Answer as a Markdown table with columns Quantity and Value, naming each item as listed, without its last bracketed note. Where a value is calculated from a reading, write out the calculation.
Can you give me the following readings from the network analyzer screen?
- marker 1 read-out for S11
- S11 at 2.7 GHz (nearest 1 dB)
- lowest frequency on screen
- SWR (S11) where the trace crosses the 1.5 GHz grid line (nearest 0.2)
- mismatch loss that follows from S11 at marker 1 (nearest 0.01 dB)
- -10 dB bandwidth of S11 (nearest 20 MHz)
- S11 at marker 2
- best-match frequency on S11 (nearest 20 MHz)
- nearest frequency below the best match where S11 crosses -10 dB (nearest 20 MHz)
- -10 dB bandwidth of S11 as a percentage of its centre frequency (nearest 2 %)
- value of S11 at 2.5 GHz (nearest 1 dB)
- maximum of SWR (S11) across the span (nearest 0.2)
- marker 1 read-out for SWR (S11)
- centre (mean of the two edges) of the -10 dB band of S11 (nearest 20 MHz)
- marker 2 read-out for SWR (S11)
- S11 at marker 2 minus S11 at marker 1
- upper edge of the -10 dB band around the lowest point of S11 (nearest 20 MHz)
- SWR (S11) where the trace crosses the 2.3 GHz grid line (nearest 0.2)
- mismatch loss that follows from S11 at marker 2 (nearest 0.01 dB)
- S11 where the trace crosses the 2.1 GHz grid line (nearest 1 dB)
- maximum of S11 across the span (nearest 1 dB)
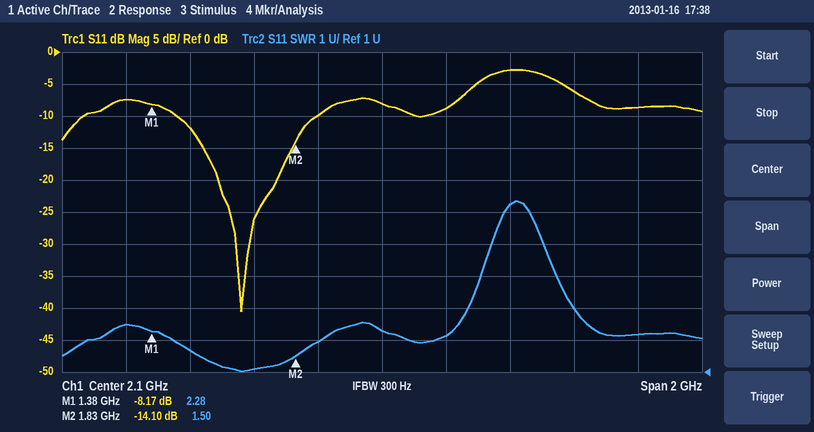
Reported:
| Quantity | Value |
|---|---|
| marker 1 read-out for S11 | -8.17 dB |
| S11 at 2.7 GHz | -6 dB |
| lowest frequency on screen | 1.1 GHz |
| SWR (S11) where the trace crosses the 1.5 GHz grid line | 1.6 |
| mismatch loss that follows from S11 at marker 1 | −10 log10(1 − 10^(-8.17/10)) ≈ 0.72 dB |
| -10 dB bandwidth of S11 | 1.90 GHz − 1.46 GHz = 440 MHz |
| S11 at marker 2 | -14.10 dB |
| best-match frequency on S11 | 1.66 GHz |
| nearest frequency below the best match where S11 crosses -10 dB | 1.46 GHz |
| -10 dB bandwidth of S11 as a percentage of its centre frequency | 440 MHz / 1.68 GHz ≈ 26 % |
| value of S11 at 2.5 GHz | -3 dB |
| maximum of SWR (S11) across the span | 6.4 |
| marker 1 read-out for SWR | 2.28 |
| centre (mean of the two edges) of the -10 dB band of S11 | 1.68 GHz |
| marker 2 read-out for SWR | 1.50 |
| S11 at marker 2 minus S11 at marker 1 | -14.1 − (-8.17) = -5.93 dB |
| upper edge of the -10 dB band around the lowest point of S11 | 1.90 GHz |
| SWR (S11) where the trace crosses the 2.3 GHz grid line | 2.2 |
| mismatch loss that follows from S11 at marker 2 | −10 log10(1 − 10^(-14.1/10)) ≈ 0.17 dB |
| S11 where the trace crosses the 2.1 GHz grid line | -8 dB |
| maximum of S11 across the span | -3 dB |
